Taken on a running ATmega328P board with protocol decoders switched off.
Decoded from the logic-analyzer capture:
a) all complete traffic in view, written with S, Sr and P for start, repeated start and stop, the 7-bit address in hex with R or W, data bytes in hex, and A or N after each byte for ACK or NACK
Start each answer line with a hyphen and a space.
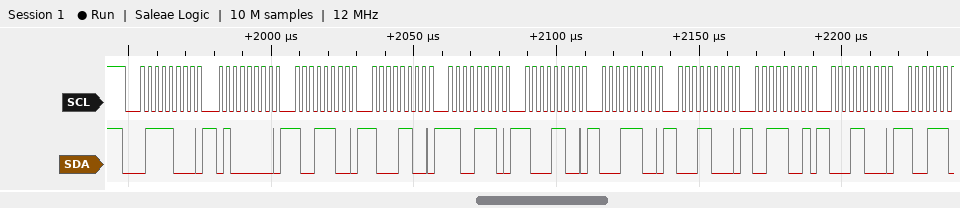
- S 3CW A 40 A 9C A 8C A CE A 8C A 1C A 18 A 39 A 18 A
